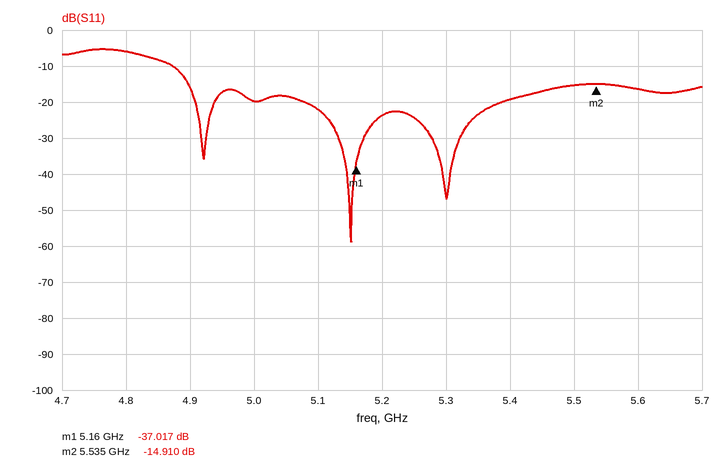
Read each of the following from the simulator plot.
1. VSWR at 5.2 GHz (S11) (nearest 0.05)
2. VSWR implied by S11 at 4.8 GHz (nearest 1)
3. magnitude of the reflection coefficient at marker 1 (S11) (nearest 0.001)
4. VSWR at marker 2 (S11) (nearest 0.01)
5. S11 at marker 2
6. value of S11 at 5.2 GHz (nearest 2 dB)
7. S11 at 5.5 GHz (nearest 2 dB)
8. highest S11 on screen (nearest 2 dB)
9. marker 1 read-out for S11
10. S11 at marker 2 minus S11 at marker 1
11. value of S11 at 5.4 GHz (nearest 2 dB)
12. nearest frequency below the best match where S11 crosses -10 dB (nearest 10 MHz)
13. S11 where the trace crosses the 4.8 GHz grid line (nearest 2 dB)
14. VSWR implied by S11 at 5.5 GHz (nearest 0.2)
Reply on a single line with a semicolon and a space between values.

1.15; 3; 0.014; 1.44; -14.910 dB; -24 dB; -16 dB; -6 dB; -37.017 dB; 22.107 dB; -20 dB; 4.87 GHz; -6 dB; 1.4
